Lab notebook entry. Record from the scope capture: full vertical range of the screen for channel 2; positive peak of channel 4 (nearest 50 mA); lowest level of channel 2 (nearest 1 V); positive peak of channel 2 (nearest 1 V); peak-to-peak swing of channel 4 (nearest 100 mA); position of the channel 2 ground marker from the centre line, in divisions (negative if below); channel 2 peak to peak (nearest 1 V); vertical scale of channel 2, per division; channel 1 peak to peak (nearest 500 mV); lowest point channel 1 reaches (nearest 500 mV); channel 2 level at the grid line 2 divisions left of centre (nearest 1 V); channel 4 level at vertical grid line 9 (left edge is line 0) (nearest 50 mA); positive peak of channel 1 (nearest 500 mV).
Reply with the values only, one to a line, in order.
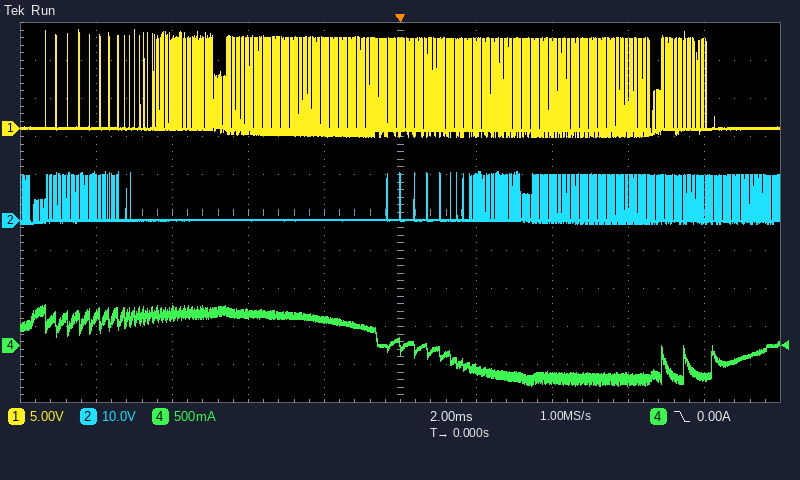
100 V
550 mA
-1 V
13 V
1.10 A
-0.2 div
14 V
10 V
14.0 V
-1.0 V
0 V
-400 mA
13.0 V
